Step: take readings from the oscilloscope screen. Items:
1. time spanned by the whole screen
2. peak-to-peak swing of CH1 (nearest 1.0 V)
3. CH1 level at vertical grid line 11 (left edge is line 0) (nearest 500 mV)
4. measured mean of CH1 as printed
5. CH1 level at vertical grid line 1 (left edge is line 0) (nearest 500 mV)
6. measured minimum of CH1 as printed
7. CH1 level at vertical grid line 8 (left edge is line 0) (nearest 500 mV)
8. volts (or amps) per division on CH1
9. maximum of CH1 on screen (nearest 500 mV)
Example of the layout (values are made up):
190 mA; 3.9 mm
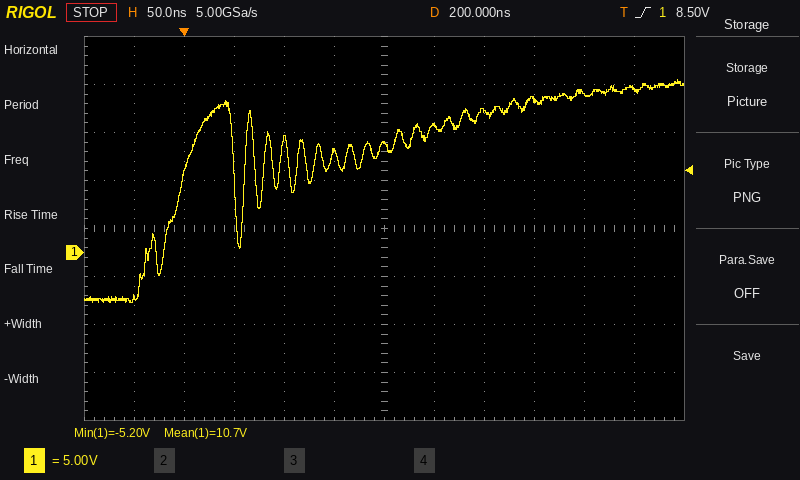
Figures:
600 ns; 23.0 V; 17.0 V; 10.7 V; -5.0 V; -5.20 V; 14.5 V; 5 V; 18.0 V
